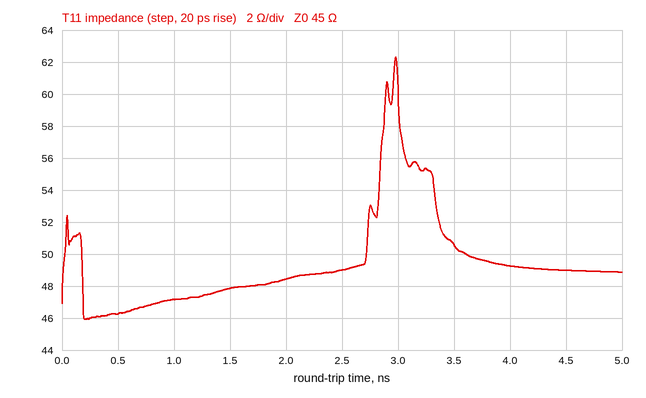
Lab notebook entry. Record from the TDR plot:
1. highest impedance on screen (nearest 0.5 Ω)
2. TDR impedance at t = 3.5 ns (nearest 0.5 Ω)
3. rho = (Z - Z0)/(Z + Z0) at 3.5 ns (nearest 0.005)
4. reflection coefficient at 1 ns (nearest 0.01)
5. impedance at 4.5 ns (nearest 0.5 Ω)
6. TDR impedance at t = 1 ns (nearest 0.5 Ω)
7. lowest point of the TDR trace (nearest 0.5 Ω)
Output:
62.5 Ω
50.5 Ω
+0.060
+0.02
49.0 Ω
47.0 Ω
46.0 Ω
